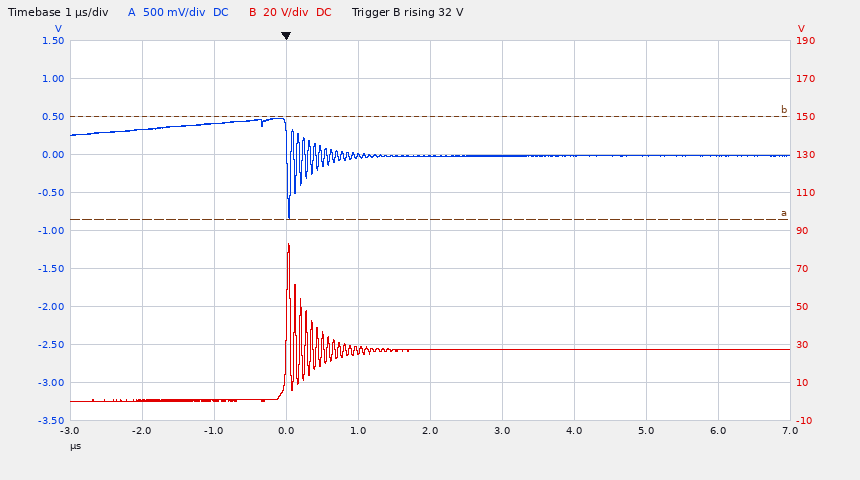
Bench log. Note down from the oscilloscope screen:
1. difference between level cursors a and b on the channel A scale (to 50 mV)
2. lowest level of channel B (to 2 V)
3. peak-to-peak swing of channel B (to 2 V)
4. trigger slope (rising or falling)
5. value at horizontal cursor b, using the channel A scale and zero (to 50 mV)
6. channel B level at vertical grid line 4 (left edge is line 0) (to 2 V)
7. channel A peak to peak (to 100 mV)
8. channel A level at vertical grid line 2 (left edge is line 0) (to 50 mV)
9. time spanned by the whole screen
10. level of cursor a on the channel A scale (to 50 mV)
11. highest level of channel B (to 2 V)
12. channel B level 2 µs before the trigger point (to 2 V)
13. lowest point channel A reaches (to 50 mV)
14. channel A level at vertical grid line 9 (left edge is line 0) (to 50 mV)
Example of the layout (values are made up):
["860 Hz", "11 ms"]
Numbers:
["1.35 V", "0 V", "84 V", "rising", "500 mV", "26 V", "1.30 V", "400 mV", "10 µs", "-850 mV", "84 V", "0 V", "-850 mV", "0 mV"]
